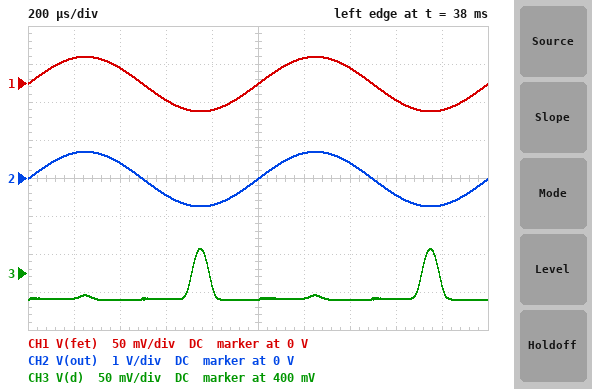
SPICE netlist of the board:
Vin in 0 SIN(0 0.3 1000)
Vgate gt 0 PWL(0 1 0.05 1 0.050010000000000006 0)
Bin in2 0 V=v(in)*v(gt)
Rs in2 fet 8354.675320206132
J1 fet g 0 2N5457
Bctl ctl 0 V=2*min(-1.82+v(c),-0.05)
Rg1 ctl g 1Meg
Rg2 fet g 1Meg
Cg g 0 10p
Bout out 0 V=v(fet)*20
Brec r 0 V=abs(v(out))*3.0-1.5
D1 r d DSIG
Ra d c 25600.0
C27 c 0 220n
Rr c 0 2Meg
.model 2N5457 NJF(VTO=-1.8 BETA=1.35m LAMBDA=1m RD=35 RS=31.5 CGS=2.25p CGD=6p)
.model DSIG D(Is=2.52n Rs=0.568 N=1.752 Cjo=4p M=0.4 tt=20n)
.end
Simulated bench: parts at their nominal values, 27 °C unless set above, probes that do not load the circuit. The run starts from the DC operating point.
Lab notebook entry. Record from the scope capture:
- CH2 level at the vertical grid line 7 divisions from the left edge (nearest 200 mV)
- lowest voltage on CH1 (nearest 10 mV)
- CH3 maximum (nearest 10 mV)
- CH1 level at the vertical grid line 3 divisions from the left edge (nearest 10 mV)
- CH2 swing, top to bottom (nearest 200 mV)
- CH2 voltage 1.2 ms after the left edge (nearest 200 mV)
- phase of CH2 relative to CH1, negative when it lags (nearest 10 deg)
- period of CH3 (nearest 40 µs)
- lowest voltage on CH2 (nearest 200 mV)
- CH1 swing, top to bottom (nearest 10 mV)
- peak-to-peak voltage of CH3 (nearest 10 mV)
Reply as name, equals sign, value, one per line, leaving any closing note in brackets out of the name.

CH2 level at the vertical grid line 7 divisions from the left edge = 400 mV
lowest voltage on CH1 = -40 mV
CH3 maximum = 430 mV
CH1 level at the vertical grid line 3 divisions from the left edge = -20 mV
CH2 swing, top to bottom = 1.4 V
CH2 voltage 1.2 ms after the left edge = 600 mV
phase of CH2 relative to CH1, negative when it lags = 0 deg
period of CH3 = 1.00 ms
lowest voltage on CH2 = -800 mV
CH1 swing, top to bottom = 70 mV
peak-to-peak voltage of CH3 = 70 mV
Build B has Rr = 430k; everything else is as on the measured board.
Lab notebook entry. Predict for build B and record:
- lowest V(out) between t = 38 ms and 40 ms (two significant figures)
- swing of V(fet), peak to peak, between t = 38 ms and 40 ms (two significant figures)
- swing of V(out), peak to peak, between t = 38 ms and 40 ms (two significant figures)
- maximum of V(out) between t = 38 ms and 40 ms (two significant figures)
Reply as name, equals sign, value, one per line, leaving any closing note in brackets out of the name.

lowest V(out) between t = 38 ms and 40 ms = -790 mV
swing of V(fet), peak to peak, between t = 38 ms and 40 ms = 76 mV
swing of V(out), peak to peak, between t = 38 ms and 40 ms = 1.5 V
maximum of V(out) between t = 38 ms and 40 ms = 730 mV
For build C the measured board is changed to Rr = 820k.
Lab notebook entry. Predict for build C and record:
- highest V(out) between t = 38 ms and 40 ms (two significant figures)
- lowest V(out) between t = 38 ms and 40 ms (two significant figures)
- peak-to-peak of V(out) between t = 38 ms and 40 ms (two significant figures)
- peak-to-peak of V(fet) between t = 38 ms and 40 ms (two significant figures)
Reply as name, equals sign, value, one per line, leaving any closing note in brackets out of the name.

highest V(out) between t = 38 ms and 40 ms = 710 mV
lowest V(out) between t = 38 ms and 40 ms = -770 mV
peak-to-peak of V(out) between t = 38 ms and 40 ms = 1.5 V
peak-to-peak of V(fet) between t = 38 ms and 40 ms = 74 mV
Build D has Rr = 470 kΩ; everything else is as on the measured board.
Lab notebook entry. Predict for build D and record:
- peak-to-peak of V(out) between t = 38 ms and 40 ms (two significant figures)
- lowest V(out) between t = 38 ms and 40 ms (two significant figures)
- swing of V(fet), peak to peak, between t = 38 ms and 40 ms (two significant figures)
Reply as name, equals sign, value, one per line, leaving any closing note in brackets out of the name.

peak-to-peak of V(out) between t = 38 ms and 40 ms = 1.5 V
lowest V(out) between t = 38 ms and 40 ms = -790 mV
swing of V(fet), peak to peak, between t = 38 ms and 40 ms = 76 mV
